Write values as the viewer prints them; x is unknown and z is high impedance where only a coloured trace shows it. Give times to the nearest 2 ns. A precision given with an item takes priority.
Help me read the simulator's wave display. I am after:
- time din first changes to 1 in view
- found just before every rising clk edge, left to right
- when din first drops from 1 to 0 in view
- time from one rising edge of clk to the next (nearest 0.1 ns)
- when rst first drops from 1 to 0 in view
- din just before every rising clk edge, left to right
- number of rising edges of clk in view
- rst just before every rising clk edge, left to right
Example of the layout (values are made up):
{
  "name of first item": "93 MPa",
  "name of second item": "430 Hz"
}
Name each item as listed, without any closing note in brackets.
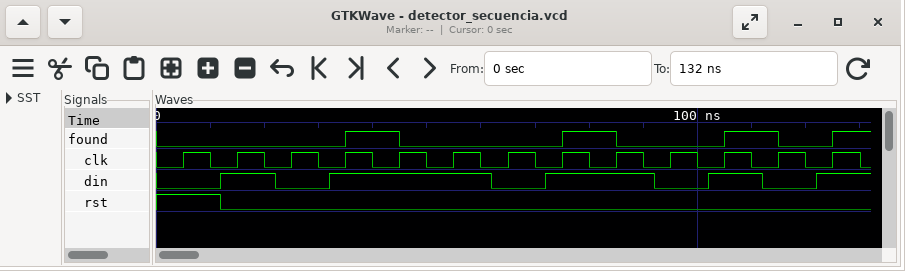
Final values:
{
  "time din first changes to 1 in view": "12 ns",
  "found just before every rising clk edge, left to right": "0 0 0 0 1 0 0 0 1 0 0 1 0",
  "when din first drops from 1 to 0 in view": "22 ns",
  "time from one rising edge of clk to the next": "10 ns",
  "when rst first drops from 1 to 0 in view": "12 ns",
  "din just before every rising clk edge, left to right": "0 1 0 1 1 1 0 1 1 0 1 0 1",
  "number of rising edges of clk in view": "13",
  "rst just before every rising clk edge, left to right": "1 0 0 0 0 0 0 0 0 0 0 0 0"
}
